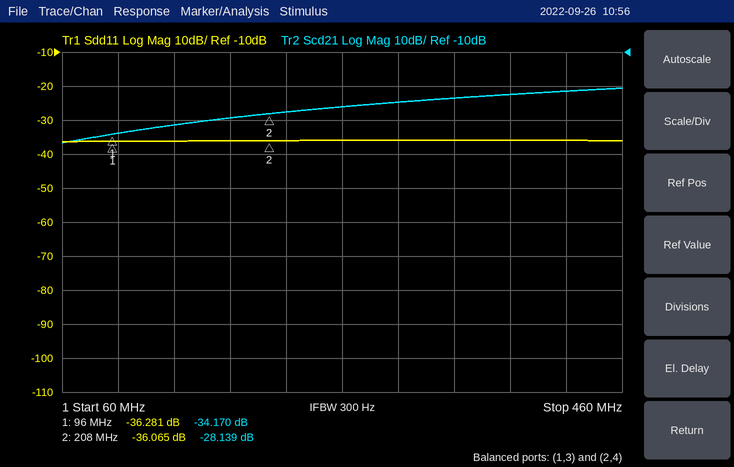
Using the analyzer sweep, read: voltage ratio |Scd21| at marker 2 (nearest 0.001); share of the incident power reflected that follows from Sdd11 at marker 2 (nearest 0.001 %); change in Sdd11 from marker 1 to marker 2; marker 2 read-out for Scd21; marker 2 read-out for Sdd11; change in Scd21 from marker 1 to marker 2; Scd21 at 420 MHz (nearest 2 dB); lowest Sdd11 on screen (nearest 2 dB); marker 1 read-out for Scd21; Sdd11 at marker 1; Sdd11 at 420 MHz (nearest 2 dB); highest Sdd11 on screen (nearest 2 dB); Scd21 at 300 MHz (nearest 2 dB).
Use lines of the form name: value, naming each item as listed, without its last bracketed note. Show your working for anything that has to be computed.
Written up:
voltage ratio |Scd21| at marker 2: 10^(-28.139/20) ≈ 0.039
share of the incident power reflected that follows from Sdd11 at marker 2: 10^(-36.065/10) ≈ 0.025 %
change in Sdd11 from marker 1 to marker 2: -36.065 − (-36.281) = 0.216 dB
marker 2 read-out for Scd21: -28.139 dB
marker 2 read-out for Sdd11: -36.065 dB
change in Scd21 from marker 1 to marker 2: -28.139 − (-34.17) = 6.031 dB
Scd21 at 420 MHz: -22 dB
lowest Sdd11 on screen: -36 dB
marker 1 read-out for Scd21: -34.170 dB
Sdd11 at marker 1: -36.281 dB
Sdd11 at 420 MHz: -36 dB
highest Sdd11 on screen: -36 dB
Scd21 at 300 MHz: -24 dB
